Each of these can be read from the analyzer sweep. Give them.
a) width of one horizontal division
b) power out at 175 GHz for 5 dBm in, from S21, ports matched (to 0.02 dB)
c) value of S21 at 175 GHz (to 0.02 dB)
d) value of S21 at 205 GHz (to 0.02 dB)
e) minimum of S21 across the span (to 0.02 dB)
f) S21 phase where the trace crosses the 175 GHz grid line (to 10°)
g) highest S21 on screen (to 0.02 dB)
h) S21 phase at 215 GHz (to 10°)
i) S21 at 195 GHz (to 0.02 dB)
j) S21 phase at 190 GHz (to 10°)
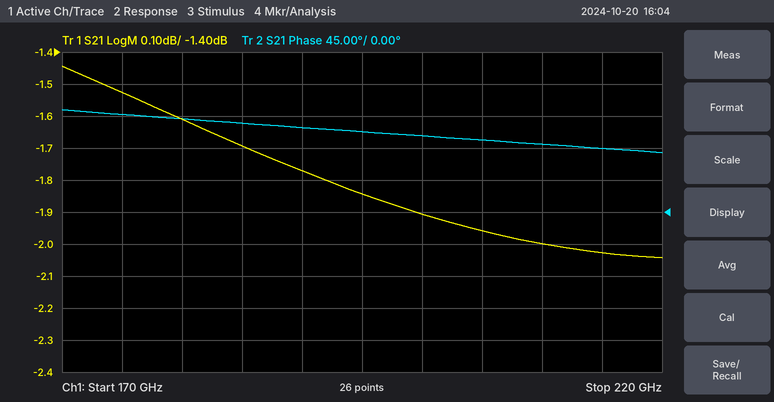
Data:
5 GHz
3.48 dBm
-1.52 dB
-1.96 dB
-2.04 dB
140°
-1.44 dB
90°
-1.84 dB
120°
